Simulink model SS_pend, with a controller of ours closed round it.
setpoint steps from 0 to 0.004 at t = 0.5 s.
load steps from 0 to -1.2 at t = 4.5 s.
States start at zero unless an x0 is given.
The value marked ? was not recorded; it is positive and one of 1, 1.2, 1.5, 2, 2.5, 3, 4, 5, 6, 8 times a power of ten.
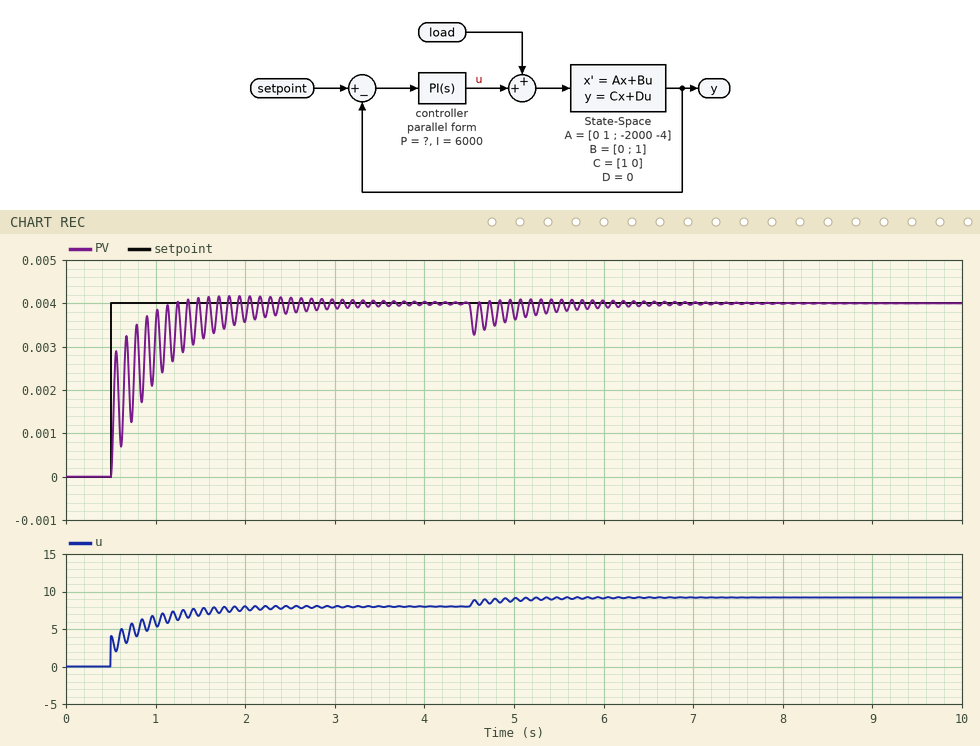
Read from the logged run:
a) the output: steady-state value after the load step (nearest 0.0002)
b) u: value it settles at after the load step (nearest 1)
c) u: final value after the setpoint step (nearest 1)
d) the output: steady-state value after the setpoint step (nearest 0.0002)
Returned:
0.0040
9
8
0.0040
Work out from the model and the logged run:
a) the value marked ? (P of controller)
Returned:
1000
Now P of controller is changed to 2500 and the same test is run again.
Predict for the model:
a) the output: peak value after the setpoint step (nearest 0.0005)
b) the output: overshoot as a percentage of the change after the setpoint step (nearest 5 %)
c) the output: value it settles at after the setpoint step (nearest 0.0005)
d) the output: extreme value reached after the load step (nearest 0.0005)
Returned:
0.0045
10 %
0.0040
0.0035
